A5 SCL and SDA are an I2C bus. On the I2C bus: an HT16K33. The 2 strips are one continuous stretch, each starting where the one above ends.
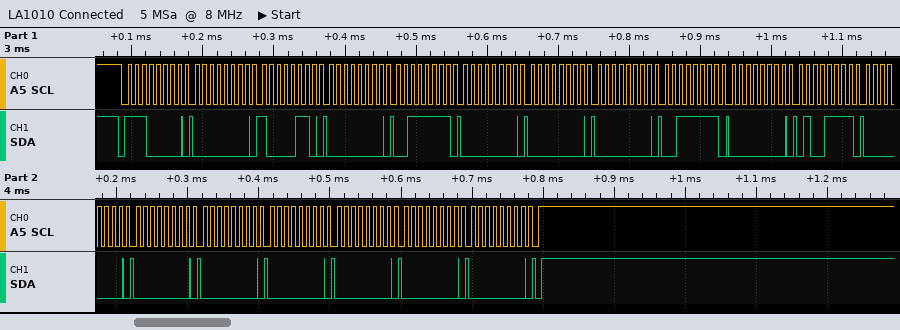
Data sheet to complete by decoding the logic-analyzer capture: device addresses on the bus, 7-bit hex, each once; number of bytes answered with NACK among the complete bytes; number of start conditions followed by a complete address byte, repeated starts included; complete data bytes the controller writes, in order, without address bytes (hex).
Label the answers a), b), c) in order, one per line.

a) 0x70
b) 0
c) 1
d) 00 86 00 3F 00 00 00 3F 00 4F 00 00 00 00 00 00 00
